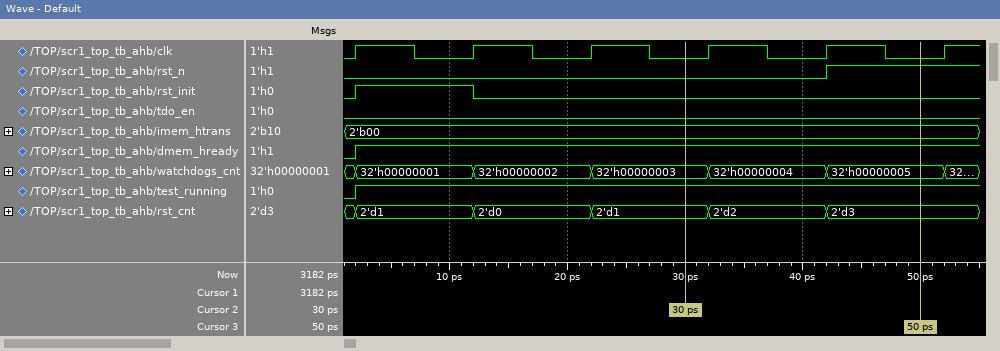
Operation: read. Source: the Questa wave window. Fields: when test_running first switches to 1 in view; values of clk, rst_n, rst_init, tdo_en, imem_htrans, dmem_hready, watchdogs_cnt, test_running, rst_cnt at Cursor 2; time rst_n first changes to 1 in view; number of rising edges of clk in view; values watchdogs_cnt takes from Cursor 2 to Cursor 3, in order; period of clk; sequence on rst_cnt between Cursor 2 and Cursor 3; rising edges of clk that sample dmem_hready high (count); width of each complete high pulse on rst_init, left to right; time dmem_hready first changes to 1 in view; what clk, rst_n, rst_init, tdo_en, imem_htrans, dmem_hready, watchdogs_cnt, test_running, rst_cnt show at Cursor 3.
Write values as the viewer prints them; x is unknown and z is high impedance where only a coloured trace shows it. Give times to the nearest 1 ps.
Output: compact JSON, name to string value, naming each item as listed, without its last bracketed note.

{"when test_running first switches to 1 in view": "2 ps", "values of clk, rst_n, rst_init, tdo_en, imem_htrans, dmem_hready, watchdogs_cnt, test_running, rst_cnt at Cursor 2": "clk=0, rst_n=0, rst_init=0, tdo_en=0, imem_htrans=2'b00, dmem_hready=1, watchdogs_cnt=32'h00000003, test_running=1, rst_cnt=2'd1", "time rst_n first changes to 1 in view": "42 ps", "number of rising edges of clk in view": "6", "values watchdogs_cnt takes from Cursor 2 to Cursor 3, in order": "32'h00000003, 32'h00000004, 32'h00000005", "period of clk": "10 ps", "sequence on rst_cnt between Cursor 2 and Cursor 3": "2'd1, 2'd2, 2'd3", "rising edges of clk that sample dmem_hready high": "5", "width of each complete high pulse on rst_init, left to right": "10 ps", "time dmem_hready first changes to 1 in view": "2 ps", "what clk, rst_n, rst_init, tdo_en, imem_htrans, dmem_hready, watchdogs_cnt, test_running, rst_cnt show at Cursor 3": "clk=0, rst_n=1, rst_init=0, tdo_en=0, imem_htrans=2'b00, dmem_hready=1, watchdogs_cnt=32'h00000005, test_running=1, rst_cnt=2'd3"}
